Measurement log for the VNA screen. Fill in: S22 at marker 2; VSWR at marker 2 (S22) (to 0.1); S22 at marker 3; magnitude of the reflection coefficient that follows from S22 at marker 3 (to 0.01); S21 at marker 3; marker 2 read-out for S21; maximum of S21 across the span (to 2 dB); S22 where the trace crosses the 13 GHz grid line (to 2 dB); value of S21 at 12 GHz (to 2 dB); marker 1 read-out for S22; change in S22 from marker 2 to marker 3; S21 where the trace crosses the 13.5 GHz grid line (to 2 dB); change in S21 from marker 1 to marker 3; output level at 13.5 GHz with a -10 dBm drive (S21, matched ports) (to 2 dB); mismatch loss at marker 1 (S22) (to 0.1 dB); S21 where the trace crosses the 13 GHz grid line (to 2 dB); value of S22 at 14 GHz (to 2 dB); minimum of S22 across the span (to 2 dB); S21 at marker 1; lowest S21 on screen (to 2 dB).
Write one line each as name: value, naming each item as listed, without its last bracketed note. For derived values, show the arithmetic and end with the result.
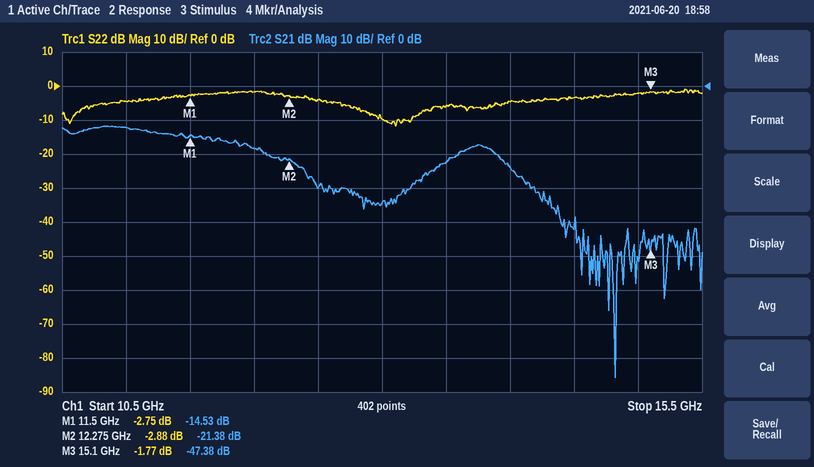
S22 at marker 2: -2.88 dB
VSWR at marker 2 (S22): (1 + 0.7178)/(1 − 0.7178) ≈ 6.1
S22 at marker 3: -1.77 dB
magnitude of the reflection coefficient that follows from S22 at marker 3: 10^(-1.77/20) ≈ 0.82
S21 at marker 3: -47.38 dB
marker 2 read-out for S21: -21.38 dB
maximum of S21 across the span: -12 dB
S22 where the trace crosses the 13 GHz grid line: -10 dB
value of S21 at 12 GHz: -18 dB
marker 1 read-out for S22: -2.75 dB
change in S22 from marker 2 to marker 3: -1.77 − (-2.88) = 1.11 dB
S21 where the trace crosses the 13.5 GHz grid line: -22 dB
change in S21 from marker 1 to marker 3: -47.38 − (-14.53) = -32.85 dB
output level at 13.5 GHz with a -10 dBm drive (S21, matched ports): -10 dBm + (-22 dB) = -32 dBm
mismatch loss at marker 1 (S22): −10 log10(1 − 10^(-2.75/10)) ≈ 3.3 dB
S21 where the trace crosses the 13 GHz grid line: -34 dB
value of S22 at 14 GHz: -4 dB
minimum of S22 across the span: -12 dB
S21 at marker 1: -14.53 dB
lowest S21 on screen: -86 dB
